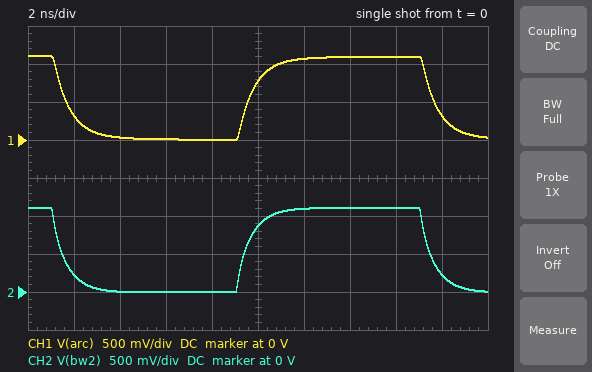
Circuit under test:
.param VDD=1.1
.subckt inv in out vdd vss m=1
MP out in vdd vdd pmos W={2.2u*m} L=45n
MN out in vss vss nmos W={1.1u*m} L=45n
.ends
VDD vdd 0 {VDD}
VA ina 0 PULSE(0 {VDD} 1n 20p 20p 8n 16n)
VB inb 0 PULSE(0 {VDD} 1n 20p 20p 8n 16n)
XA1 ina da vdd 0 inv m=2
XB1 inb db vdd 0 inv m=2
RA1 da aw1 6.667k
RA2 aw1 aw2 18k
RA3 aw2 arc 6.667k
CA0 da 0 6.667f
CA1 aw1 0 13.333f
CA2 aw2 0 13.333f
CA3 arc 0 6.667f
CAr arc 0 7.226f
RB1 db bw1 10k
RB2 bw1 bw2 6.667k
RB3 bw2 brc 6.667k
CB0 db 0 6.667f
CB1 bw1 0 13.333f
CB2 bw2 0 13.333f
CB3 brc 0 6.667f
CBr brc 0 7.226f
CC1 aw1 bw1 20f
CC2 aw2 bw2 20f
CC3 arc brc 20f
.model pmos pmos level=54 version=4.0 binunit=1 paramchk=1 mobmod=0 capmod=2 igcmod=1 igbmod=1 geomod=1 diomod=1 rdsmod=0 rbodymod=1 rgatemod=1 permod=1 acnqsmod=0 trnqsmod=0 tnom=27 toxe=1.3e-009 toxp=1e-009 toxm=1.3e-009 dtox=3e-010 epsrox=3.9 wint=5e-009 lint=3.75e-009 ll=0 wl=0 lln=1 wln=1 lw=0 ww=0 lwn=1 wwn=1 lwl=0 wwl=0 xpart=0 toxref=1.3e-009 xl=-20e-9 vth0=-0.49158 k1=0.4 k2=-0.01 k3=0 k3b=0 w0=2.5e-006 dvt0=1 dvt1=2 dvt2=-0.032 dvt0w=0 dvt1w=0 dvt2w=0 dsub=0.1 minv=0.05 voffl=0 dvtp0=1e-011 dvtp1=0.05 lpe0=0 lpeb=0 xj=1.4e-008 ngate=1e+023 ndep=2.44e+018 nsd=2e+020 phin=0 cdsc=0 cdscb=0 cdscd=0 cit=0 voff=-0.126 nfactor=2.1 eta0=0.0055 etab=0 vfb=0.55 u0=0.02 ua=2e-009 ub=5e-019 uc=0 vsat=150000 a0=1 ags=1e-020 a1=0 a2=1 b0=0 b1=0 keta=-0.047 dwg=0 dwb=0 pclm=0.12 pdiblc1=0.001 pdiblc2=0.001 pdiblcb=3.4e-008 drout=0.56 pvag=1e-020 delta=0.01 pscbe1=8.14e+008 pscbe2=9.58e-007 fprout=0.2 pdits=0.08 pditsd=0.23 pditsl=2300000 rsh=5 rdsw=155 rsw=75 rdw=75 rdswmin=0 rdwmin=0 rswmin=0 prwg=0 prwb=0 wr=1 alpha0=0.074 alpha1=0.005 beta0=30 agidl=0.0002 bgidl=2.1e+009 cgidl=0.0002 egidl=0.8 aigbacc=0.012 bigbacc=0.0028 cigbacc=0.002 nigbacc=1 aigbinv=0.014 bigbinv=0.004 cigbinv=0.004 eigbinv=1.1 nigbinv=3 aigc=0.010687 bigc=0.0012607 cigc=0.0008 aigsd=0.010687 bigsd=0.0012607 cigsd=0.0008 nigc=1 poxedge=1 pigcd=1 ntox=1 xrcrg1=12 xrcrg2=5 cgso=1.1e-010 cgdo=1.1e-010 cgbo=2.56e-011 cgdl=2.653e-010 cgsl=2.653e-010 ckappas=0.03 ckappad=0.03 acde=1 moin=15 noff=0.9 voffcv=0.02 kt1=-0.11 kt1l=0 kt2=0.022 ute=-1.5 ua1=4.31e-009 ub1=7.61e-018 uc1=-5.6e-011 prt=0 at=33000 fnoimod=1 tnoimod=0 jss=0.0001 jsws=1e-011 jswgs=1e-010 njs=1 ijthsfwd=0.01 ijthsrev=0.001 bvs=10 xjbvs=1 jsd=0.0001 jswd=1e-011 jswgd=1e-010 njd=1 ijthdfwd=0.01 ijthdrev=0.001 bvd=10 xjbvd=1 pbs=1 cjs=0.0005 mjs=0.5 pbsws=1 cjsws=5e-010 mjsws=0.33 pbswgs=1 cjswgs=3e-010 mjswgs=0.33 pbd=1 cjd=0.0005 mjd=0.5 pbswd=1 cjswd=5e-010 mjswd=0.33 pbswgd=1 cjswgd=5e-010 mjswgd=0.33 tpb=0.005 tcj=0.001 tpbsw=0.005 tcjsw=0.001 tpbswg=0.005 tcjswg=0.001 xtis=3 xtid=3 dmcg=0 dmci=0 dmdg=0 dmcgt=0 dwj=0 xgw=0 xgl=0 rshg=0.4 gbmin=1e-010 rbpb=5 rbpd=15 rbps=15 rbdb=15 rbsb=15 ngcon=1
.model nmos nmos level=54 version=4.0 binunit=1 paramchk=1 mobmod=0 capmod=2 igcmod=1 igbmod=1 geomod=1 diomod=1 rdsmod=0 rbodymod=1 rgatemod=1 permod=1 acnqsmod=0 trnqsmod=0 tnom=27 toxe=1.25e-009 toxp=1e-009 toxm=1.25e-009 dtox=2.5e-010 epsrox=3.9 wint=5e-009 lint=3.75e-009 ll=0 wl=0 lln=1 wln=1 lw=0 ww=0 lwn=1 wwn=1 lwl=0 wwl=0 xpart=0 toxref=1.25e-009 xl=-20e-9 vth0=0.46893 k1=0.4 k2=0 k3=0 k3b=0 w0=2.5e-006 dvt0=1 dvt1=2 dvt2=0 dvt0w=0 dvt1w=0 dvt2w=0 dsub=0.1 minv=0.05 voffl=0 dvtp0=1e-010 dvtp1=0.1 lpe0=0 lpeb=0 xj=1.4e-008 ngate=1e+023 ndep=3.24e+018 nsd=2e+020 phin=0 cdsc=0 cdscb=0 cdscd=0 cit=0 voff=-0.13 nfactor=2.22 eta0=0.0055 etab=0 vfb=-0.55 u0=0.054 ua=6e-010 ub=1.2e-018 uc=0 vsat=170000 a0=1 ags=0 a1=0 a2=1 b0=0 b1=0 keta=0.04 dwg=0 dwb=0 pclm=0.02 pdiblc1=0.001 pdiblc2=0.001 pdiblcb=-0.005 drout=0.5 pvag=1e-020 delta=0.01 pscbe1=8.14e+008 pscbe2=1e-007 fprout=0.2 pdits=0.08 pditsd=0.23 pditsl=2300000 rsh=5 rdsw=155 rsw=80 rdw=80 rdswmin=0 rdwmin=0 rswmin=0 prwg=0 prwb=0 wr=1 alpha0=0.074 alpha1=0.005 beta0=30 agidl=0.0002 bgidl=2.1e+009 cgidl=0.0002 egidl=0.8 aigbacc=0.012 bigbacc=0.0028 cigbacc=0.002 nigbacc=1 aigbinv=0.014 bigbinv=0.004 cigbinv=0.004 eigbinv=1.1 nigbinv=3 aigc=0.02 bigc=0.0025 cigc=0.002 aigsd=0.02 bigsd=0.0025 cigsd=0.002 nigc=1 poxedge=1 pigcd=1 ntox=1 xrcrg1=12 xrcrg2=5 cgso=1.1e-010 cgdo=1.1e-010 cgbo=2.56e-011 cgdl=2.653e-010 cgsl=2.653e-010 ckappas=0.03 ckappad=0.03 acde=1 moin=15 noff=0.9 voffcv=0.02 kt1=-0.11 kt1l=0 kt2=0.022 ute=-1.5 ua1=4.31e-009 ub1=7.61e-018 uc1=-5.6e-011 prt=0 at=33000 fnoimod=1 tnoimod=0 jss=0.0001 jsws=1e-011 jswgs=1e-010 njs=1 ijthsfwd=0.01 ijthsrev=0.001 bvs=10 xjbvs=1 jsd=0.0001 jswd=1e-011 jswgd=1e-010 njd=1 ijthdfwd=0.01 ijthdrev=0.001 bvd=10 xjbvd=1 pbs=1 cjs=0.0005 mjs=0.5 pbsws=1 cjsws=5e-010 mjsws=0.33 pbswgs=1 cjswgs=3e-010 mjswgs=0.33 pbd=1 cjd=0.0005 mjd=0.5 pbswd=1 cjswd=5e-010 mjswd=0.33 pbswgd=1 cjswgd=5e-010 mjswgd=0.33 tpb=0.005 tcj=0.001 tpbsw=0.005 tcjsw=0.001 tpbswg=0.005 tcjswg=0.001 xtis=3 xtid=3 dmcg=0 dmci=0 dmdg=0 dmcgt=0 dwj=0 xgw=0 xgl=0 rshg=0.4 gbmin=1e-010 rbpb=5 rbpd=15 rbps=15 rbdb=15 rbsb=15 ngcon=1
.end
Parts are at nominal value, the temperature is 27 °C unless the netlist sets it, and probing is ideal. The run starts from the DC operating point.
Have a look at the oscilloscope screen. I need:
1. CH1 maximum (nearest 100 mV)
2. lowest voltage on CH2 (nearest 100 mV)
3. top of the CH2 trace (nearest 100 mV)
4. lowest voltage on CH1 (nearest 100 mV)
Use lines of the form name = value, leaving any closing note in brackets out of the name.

CH1 maximum = 1.1 V
lowest voltage on CH2 = 0 V
top of the CH2 trace = 1.1 V
lowest voltage on CH1 = 0 V
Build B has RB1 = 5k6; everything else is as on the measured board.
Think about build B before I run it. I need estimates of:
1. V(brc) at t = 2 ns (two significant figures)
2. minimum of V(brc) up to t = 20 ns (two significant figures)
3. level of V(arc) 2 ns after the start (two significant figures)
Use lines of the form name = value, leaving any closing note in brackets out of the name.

V(brc) at t = 2 ns = 170 mV
minimum of V(brc) up to t = 20 ns = -15 mV
level of V(arc) 2 ns after the start = 280 mV
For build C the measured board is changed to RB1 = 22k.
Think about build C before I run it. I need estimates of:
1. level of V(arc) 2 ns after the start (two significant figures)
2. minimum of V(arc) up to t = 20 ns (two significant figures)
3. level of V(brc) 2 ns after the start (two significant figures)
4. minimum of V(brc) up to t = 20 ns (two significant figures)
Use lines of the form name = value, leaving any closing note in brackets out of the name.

level of V(arc) 2 ns after the start = 390 mV
minimum of V(arc) up to t = 20 ns = -11 mV
level of V(brc) 2 ns after the start = 410 mV
minimum of V(brc) up to t = 20 ns = 11 mV
